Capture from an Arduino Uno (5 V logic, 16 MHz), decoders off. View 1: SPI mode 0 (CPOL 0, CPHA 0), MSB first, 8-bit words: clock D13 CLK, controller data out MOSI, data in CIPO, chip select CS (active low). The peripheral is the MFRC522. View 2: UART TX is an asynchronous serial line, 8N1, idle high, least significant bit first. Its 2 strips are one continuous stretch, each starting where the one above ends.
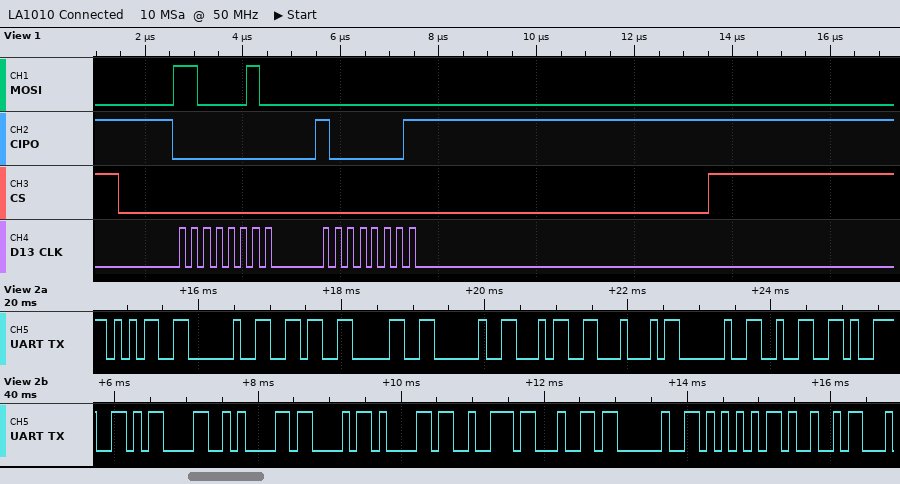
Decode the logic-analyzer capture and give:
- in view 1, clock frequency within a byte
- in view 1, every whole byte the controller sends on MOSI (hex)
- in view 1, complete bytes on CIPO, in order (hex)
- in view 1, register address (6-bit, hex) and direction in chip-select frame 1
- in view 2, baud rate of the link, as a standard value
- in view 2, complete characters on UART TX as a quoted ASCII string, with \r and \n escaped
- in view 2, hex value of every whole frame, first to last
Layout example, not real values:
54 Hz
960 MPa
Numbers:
4 MHz
0xC2 0x00
0x00 0x81
0x21 read
9600 baud
"5 60 4D 29\r\nCard UI"
0x35 0x20 0x36 0x30 0x20 0x34 0x44 0x20 0x32 0x39 0x0D 0x0A 0x43 0x61 0x72 0x64 0x20 0x55 0x49
